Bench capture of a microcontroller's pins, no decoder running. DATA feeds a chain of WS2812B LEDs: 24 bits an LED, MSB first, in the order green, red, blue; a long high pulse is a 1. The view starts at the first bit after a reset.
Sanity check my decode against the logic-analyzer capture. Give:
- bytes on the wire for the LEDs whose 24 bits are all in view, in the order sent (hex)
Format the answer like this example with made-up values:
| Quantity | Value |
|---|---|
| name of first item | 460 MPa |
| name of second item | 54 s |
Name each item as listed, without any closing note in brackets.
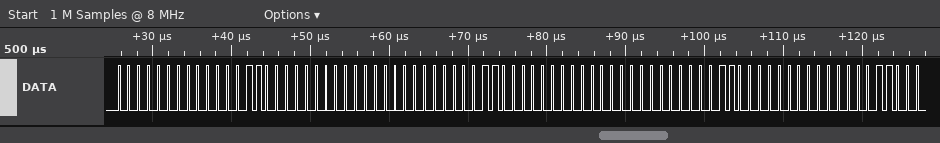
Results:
| Quantity | Value |
|---|---|
| bytes on the wire for the LEDs whose 24 bits are all in view, in the order sent | 00 06 00 00 06 00 00 06 00 |
